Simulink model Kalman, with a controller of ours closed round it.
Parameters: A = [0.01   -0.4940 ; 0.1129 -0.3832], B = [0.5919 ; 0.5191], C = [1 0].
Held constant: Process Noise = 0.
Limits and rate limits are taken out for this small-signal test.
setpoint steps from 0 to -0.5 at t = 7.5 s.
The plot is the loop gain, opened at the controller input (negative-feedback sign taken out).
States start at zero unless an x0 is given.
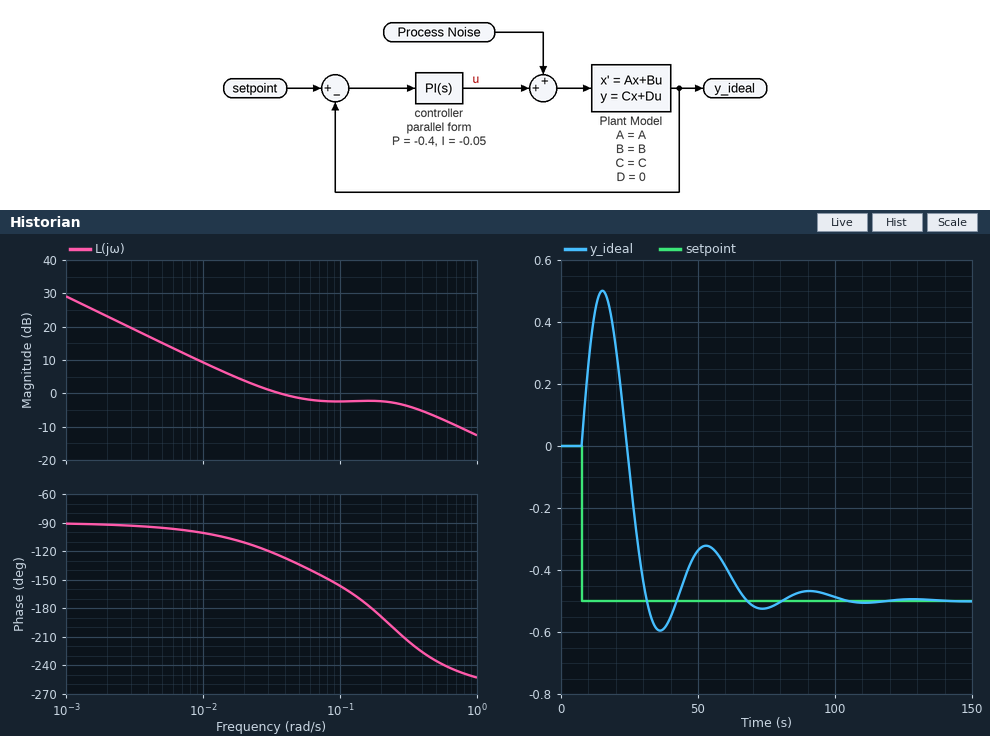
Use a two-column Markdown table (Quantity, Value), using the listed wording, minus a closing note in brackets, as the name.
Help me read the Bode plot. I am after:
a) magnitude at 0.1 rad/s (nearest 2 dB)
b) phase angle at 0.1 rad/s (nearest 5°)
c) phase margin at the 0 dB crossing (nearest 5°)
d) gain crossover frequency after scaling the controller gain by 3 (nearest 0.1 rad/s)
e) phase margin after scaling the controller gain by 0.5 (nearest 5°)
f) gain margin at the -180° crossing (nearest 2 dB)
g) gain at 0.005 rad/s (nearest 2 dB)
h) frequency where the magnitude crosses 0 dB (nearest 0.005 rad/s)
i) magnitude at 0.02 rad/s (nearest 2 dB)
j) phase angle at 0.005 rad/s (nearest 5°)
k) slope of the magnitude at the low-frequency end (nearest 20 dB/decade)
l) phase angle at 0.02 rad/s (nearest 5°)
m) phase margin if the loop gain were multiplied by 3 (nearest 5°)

| Quantity | Value |
|---|---|
| magnitude at 0.1 rad/s | -2 dB |
| phase angle at 0.1 rad/s | -155° |
| phase margin at the 0 dB crossing | 55° |
| gain crossover frequency after scaling the controller gain by 3 | 0.7 rad/s |
| phase margin after scaling the controller gain by 0.5 | 75° |
| gain margin at the -180° crossing | 2 dB |
| gain at 0.005 rad/s | 16 dB |
| frequency where the magnitude crosses 0 dB | 0.035 rad/s |
| magnitude at 0.02 rad/s | 4 dB |
| phase angle at 0.005 rad/s | -95° |
| slope of the magnitude at the low-frequency end | -20 dB/decade |
| phase angle at 0.02 rad/s | -110° |
| phase margin if the loop gain were multiplied by 3 | -65° |
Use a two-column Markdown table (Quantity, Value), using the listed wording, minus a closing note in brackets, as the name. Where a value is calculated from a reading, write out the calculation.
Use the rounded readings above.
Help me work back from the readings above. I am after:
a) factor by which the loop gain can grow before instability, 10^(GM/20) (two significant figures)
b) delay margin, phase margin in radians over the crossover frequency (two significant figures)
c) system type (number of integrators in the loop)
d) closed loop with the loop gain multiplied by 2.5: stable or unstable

| Quantity | Value |
|---|---|
| factor by which the loop gain can grow before instability, 10^(GM/20) | 10^(2 / 20) = 1.3 |
| delay margin, phase margin in radians over the crossover frequency | 55 × π / 180 / 0.035 = 27 s |
| system type | 1 |
| closed loop with the loop gain multiplied by 2.5: stable or unstable | unstable |
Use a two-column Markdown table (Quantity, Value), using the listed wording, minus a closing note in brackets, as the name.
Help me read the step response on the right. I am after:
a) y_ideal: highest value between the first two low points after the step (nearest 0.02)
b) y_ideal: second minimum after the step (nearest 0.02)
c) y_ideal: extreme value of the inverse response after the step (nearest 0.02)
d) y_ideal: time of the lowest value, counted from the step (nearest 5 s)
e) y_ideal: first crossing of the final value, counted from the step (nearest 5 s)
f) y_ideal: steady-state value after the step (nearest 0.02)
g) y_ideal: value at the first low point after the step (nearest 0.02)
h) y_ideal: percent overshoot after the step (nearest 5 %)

| Quantity | Value |
|---|---|
| y_ideal: highest value between the first two low points after the step | -0.32 |
| y_ideal: second minimum after the step | -0.52 |
| y_ideal: extreme value of the inverse response after the step | 0.50 |
| y_ideal: time of the lowest value, counted from the step | 30 s |
| y_ideal: first crossing of the final value, counted from the step | 25 s |
| y_ideal: steady-state value after the step | -0.50 |
| y_ideal: value at the first low point after the step | -0.60 |
| y_ideal: percent overshoot after the step | 20 % |
